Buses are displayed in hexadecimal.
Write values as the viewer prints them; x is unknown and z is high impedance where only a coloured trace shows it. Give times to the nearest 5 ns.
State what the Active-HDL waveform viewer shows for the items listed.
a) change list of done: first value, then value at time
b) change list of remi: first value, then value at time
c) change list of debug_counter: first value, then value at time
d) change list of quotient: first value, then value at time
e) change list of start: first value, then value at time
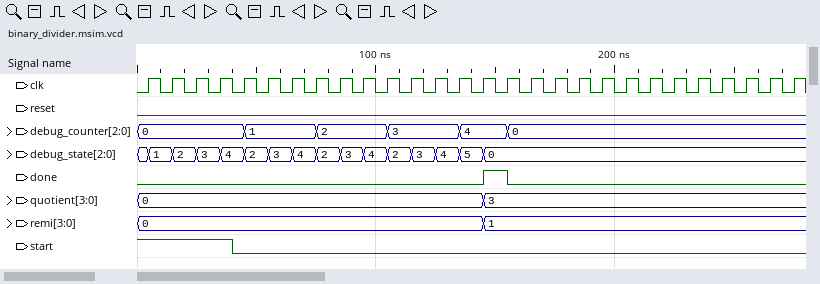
0, 1 at 145 ns, 0 at 155 ns
0, 1 at 145 ns
0, 1 at 45 ns, 2 at 75 ns, 3 at 105 ns, 4 at 135 ns, 0 at 155 ns
0, 3 at 145 ns
1, 0 at 40 ns
